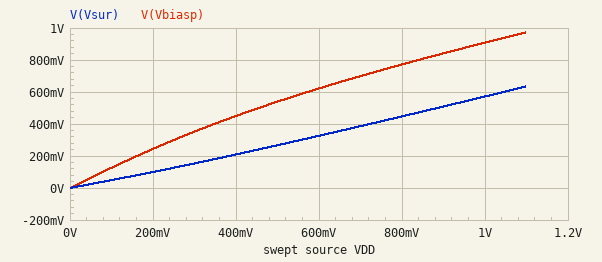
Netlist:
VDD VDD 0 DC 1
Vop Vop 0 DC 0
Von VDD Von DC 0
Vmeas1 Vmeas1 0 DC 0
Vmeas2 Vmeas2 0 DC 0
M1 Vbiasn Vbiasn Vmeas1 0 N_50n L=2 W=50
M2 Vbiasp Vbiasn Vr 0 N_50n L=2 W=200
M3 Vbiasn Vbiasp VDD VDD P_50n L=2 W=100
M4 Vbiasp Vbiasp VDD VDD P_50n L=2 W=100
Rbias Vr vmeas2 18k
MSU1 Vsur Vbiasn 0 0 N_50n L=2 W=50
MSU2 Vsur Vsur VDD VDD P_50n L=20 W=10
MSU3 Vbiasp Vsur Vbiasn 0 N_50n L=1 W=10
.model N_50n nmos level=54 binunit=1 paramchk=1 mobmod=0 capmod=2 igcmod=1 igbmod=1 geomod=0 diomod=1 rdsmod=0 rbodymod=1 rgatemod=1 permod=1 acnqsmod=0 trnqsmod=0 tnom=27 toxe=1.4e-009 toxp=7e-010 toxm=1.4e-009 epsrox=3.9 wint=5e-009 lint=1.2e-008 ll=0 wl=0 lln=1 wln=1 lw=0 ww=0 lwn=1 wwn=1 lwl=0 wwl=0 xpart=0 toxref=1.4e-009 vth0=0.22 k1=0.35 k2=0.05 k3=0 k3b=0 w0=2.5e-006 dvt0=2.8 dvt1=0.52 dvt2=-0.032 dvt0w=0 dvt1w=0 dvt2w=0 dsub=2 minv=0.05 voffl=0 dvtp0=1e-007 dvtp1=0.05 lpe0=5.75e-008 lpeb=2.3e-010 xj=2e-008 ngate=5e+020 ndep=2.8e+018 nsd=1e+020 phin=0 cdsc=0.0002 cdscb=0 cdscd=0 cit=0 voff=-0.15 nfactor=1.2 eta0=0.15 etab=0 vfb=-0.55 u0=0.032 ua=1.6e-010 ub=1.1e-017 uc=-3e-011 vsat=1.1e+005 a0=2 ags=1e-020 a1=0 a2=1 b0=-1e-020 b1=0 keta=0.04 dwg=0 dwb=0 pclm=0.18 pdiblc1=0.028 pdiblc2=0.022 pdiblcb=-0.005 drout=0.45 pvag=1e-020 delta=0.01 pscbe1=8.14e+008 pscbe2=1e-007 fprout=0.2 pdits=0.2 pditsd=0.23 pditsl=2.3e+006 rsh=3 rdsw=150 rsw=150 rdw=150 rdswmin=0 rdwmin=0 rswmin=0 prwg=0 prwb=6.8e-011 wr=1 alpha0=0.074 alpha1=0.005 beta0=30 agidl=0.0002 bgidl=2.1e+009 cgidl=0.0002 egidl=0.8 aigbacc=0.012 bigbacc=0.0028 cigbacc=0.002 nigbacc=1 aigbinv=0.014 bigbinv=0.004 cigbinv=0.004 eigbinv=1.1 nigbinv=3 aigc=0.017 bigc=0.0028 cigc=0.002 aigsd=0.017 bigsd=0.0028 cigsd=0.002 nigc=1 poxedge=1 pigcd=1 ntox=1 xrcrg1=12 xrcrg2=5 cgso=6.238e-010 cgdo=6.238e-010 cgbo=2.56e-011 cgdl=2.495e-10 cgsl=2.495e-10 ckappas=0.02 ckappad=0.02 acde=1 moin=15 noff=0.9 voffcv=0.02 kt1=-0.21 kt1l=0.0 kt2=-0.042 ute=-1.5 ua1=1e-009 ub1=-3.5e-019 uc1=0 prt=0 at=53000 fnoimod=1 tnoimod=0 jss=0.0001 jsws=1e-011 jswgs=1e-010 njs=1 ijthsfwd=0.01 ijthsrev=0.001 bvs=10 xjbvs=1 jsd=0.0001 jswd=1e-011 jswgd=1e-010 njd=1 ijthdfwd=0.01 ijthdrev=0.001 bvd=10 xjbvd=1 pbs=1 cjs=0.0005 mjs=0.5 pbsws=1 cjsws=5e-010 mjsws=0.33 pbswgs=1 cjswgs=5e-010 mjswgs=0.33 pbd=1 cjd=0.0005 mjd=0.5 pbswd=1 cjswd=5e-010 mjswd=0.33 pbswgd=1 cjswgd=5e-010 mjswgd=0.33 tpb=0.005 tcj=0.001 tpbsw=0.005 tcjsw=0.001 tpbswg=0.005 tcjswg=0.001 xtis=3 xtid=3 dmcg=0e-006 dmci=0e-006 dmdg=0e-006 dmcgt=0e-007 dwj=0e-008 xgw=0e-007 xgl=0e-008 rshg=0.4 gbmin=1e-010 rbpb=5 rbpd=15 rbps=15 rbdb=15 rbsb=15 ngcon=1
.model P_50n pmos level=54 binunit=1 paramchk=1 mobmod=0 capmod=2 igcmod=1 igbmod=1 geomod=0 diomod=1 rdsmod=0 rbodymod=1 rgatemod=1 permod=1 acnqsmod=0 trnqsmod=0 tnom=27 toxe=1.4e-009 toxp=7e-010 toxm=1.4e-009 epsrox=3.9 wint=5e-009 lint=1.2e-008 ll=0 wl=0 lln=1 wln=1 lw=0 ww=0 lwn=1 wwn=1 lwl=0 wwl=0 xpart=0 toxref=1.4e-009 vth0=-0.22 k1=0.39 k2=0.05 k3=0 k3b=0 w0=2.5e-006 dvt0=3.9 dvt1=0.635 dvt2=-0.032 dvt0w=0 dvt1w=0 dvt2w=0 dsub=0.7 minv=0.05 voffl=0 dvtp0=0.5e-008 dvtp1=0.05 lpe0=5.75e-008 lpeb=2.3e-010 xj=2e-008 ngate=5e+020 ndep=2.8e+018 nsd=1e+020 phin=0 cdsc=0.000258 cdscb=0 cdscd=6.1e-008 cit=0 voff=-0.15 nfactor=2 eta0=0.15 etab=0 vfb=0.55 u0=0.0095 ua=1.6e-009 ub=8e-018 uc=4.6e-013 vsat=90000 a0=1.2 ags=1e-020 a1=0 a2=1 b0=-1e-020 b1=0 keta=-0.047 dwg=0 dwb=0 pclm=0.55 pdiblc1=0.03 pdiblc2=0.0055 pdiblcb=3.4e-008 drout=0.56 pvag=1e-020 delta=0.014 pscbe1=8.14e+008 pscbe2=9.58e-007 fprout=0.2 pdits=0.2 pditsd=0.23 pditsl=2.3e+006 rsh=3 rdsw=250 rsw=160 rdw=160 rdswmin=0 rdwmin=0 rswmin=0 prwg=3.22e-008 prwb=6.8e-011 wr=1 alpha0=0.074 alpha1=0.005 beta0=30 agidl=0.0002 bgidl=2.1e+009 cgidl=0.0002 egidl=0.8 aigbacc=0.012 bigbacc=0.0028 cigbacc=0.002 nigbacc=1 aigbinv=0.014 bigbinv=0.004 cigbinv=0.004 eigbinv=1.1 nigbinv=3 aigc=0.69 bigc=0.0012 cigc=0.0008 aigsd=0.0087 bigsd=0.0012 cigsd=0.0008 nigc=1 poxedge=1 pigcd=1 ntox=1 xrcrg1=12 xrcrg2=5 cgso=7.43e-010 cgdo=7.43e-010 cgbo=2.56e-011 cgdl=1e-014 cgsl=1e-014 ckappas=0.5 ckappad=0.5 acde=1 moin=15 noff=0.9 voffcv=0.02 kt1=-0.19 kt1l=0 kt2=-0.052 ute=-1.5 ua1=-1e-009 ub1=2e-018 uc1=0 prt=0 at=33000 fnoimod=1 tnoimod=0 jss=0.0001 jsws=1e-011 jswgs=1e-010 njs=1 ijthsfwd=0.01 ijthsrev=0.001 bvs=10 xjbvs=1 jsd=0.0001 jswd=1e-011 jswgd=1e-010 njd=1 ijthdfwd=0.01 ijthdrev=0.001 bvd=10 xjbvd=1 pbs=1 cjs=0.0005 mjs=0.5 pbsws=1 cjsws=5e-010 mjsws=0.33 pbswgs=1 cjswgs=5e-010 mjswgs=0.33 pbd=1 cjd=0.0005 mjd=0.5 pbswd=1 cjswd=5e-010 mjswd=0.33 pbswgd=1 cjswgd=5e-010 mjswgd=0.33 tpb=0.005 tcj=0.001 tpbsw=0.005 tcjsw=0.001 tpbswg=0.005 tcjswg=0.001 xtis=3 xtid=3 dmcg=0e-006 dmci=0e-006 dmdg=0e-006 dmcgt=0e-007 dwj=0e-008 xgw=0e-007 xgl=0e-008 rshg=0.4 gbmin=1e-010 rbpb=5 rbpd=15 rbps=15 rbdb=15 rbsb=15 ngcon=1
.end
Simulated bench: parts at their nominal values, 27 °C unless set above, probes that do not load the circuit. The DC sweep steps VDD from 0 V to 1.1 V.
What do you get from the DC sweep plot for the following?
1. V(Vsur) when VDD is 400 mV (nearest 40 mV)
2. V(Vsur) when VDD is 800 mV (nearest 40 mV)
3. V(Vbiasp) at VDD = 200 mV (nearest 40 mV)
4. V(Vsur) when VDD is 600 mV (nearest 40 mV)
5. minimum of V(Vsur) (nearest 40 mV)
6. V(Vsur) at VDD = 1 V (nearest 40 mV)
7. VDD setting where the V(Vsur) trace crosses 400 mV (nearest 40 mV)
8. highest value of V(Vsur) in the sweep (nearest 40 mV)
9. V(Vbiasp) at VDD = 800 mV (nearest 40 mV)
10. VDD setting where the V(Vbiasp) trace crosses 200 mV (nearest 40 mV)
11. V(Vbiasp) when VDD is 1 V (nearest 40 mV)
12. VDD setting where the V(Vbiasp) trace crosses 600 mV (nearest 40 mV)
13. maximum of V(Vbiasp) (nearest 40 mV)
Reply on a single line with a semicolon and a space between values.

200 mV; 440 mV; 240 mV; 320 mV; 0 V; 560 mV; 720 mV; 640 mV; 760 mV; 160 mV; 920 mV; 560 mV; 960 mV
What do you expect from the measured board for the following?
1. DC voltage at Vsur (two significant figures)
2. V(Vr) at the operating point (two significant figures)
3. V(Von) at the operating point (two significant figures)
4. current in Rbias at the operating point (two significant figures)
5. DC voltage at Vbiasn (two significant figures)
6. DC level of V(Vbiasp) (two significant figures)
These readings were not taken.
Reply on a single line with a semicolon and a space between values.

570 mV; 220 mV; 1.0 V; 12 µA; 320 mV; 910 mV
